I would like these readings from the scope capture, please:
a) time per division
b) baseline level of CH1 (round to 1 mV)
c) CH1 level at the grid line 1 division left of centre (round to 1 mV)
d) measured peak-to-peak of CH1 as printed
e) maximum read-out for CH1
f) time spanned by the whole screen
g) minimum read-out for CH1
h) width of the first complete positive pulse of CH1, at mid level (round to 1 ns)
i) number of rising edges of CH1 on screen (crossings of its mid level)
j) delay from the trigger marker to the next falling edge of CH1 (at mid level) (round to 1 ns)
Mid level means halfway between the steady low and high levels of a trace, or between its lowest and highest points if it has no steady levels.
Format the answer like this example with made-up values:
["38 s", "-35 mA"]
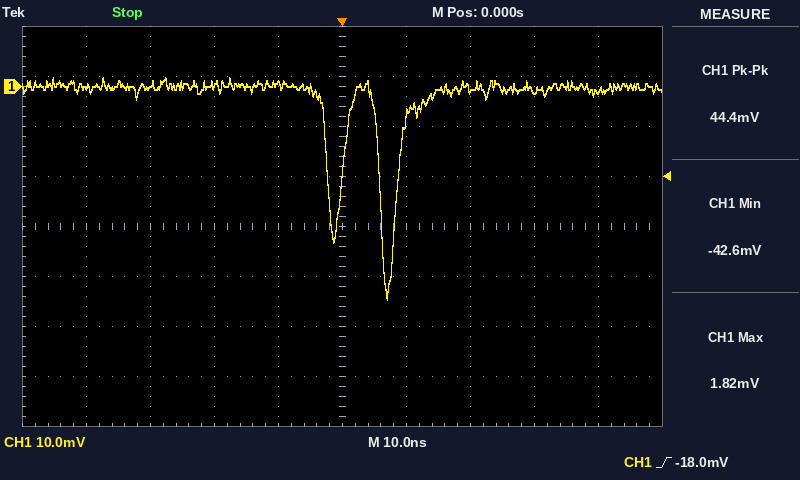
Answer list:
["10 ns", "0 mV", "0 mV", "44.4 mV", "1.82 mV", "100 ns", "-42.6 mV", "6 ns", "2", "6 ns"]
